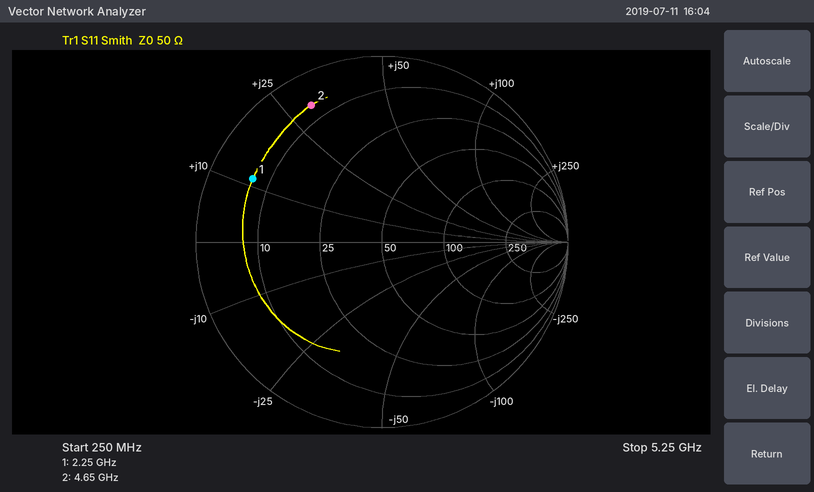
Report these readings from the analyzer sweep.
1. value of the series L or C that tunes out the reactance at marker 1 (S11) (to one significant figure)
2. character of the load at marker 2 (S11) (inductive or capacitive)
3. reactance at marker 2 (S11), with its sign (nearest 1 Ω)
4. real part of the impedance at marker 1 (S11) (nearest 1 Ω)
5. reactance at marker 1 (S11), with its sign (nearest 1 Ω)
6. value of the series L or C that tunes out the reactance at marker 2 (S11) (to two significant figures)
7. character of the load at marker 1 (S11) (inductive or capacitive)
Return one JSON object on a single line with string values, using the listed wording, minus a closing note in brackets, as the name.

{"value of the series L or C that tunes out the reactance at marker 1 (S11)": "6 pF", "character of the load at marker 2 (S11)": "inductive", "reactance at marker 2 (S11), with its sign": "+30 Ω", "real part of the impedance at marker 1 (S11)": "7 Ω", "reactance at marker 1 (S11), with its sign": "+11 Ω", "value of the series L or C that tunes out the reactance at marker 2 (S11)": "1.1 pF", "character of the load at marker 1 (S11)": "inductive"}
